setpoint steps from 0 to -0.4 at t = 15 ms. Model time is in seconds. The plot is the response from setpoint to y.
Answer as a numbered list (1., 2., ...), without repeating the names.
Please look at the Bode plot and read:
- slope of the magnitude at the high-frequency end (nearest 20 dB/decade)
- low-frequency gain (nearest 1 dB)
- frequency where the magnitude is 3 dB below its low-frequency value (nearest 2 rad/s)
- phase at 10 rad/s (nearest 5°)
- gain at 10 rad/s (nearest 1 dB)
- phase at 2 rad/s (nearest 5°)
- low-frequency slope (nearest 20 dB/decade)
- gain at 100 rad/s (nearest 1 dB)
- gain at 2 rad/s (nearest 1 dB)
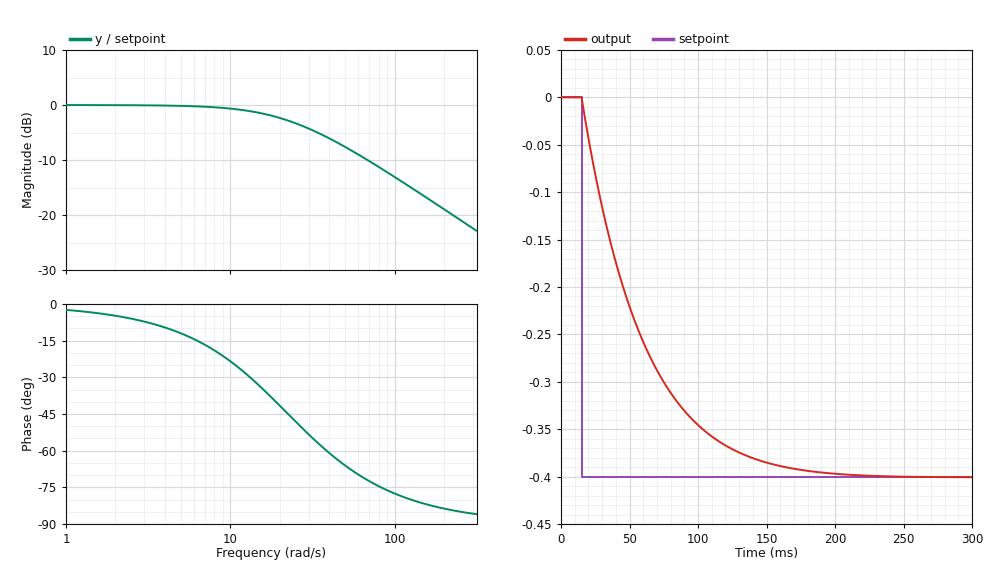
1. -20 dB/decade
2. 0 dB
3. 24 rad/s
4. -25°
5. -1 dB
6. -5°
7. 0 dB/decade
8. -13 dB
9. 0 dB
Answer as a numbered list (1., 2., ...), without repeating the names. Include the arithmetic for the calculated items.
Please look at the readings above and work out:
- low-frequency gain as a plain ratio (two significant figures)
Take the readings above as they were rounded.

1. 10^(0 / 20) = 1.0
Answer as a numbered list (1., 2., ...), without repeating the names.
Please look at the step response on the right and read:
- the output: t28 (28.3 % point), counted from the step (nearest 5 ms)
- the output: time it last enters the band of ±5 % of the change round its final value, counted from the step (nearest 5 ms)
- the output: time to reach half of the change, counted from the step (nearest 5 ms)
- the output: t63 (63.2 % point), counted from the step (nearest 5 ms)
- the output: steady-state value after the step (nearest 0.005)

1. 15 ms
2. 125 ms
3. 30 ms
4. 45 ms
5. -0.400
